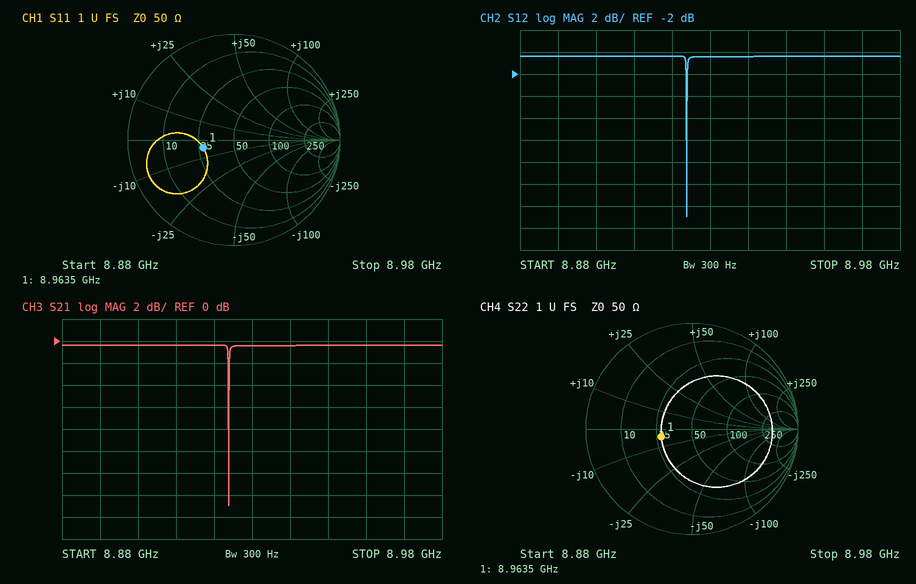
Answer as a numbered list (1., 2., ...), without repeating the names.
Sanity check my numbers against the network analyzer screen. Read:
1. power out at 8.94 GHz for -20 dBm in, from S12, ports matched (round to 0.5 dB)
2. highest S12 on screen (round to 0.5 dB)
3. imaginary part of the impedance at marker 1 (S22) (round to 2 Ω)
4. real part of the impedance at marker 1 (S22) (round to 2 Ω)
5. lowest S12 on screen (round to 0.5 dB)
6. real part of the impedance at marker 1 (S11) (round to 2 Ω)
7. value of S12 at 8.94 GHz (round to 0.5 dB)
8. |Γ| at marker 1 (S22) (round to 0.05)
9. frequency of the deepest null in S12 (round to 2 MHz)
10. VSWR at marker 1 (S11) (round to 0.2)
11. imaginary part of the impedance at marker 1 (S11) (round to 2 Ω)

1. -20.5 dBm
2. -0.5 dB
3. -4 Ω
4. 28 Ω
5. -15.0 dB
6. 28 Ω
7. -0.5 dB
8. 0.30
9. 8.924 GHz
10. 1.8
11. -4 Ω
